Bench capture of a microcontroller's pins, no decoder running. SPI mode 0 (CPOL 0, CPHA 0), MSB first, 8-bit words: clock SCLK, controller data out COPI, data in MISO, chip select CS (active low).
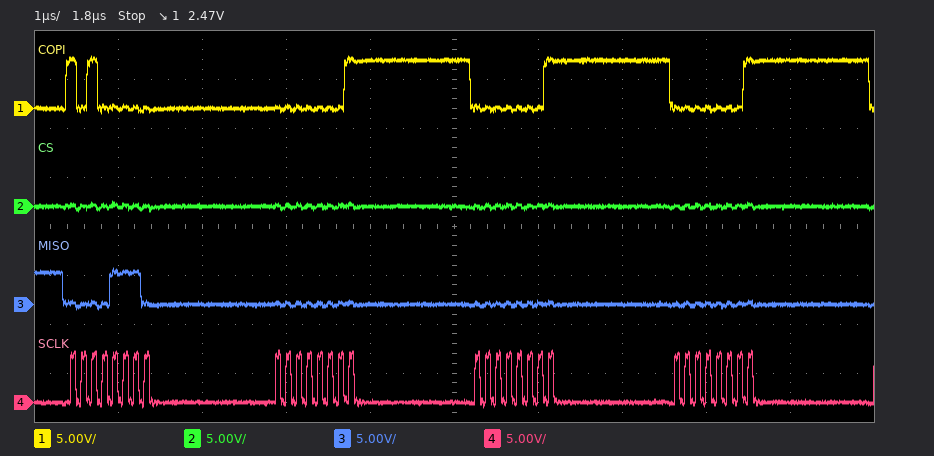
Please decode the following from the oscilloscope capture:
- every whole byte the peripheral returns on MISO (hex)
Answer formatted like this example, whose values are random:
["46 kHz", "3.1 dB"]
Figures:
["0E 00 00 00"]
